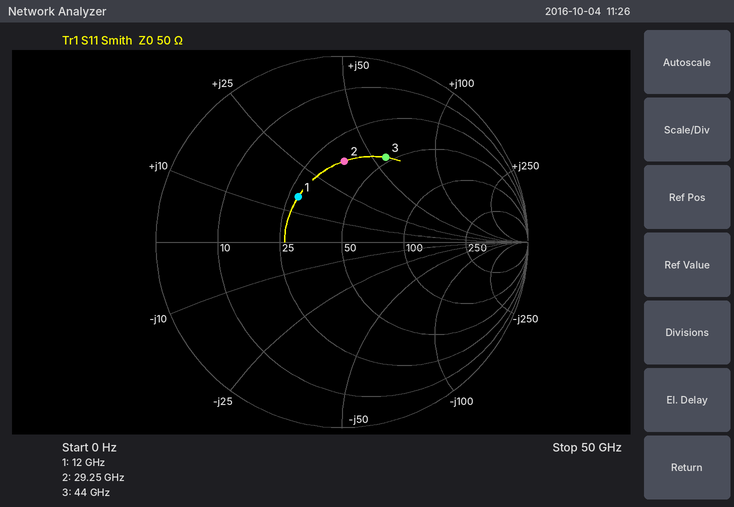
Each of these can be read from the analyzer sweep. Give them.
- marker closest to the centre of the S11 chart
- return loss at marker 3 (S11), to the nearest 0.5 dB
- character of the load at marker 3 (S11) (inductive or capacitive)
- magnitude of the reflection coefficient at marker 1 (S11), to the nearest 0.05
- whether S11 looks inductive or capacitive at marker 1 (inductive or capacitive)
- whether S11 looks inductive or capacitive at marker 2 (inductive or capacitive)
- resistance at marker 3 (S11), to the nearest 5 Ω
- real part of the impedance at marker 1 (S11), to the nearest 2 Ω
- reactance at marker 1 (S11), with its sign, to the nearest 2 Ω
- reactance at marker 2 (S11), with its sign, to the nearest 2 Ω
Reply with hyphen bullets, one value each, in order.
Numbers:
- marker 1
- 6.0 dB
- inductive
- 0.35
- inductive
- inductive
- 45 Ω
- 28 Ω
- +16 Ω
- +38 Ω
